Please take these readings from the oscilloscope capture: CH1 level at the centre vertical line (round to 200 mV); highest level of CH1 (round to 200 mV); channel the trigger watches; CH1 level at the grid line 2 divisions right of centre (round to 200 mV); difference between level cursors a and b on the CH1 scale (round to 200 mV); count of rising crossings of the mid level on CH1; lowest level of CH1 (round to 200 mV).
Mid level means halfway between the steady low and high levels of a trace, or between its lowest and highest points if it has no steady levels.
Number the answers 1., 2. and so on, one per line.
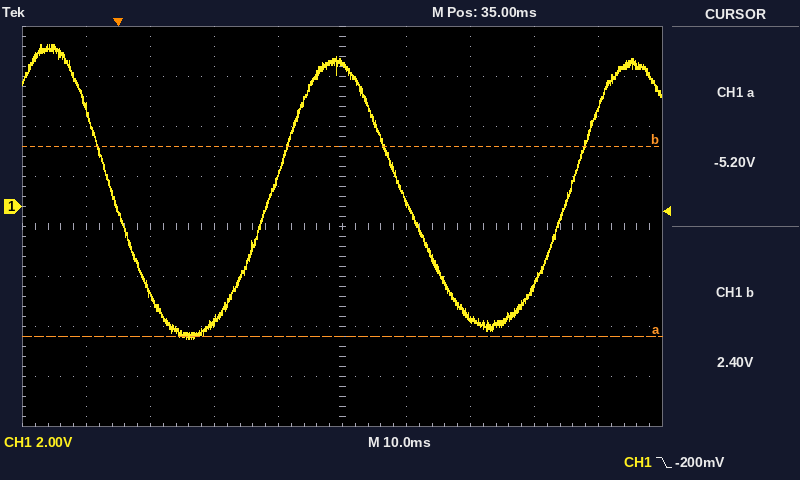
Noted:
1. 5.8 V
2. 6.4 V
3. CH1
4. -4.4 V
5. 7.6 V
6. 2
7. -5.2 V
